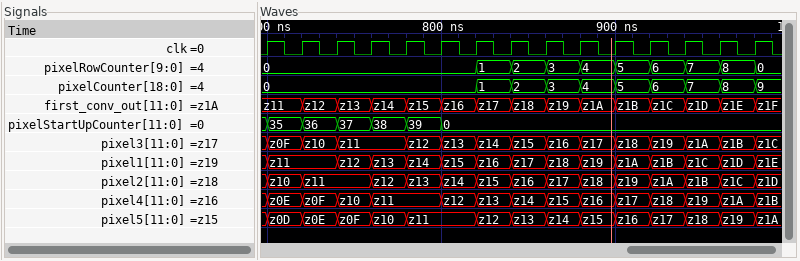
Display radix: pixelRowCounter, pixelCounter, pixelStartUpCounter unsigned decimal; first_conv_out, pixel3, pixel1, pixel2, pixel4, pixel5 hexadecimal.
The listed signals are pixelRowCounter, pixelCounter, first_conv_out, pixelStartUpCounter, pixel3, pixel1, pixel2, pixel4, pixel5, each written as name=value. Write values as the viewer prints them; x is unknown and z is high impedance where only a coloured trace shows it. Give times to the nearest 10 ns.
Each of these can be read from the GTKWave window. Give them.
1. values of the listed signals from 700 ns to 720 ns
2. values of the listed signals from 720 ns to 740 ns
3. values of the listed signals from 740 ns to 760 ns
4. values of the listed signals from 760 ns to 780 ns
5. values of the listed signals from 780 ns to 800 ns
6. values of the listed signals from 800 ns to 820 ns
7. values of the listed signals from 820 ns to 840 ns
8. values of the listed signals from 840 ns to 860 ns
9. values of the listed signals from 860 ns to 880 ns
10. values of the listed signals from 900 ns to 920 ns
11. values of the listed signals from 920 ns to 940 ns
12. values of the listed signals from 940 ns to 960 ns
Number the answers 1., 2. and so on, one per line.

1. pixelRowCounter=0, pixelCounter=0, first_conv_out=z11, pixelStartUpCounter=35, pixel3=z0F, pixel1=z11, pixel2=z10, pixel4=z0E, pixel5=z0D
2. pixelRowCounter=0, pixelCounter=0, first_conv_out=z12, pixelStartUpCounter=36, pixel3=z10, pixel1=z11, pixel2=z11, pixel4=z0F, pixel5=z0E
3. pixelRowCounter=0, pixelCounter=0, first_conv_out=z13, pixelStartUpCounter=37, pixel3=z11, pixel1=z12, pixel2=z11, pixel4=z10, pixel5=z0F
4. pixelRowCounter=0, pixelCounter=0, first_conv_out=z14, pixelStartUpCounter=38, pixel3=z11, pixel1=z13, pixel2=z12, pixel4=z11, pixel5=z10
5. pixelRowCounter=0, pixelCounter=0, first_conv_out=z15, pixelStartUpCounter=39, pixel3=z12, pixel1=z14, pixel2=z13, pixel4=z11, pixel5=z11
6. pixelRowCounter=0, pixelCounter=0, first_conv_out=z16, pixelStartUpCounter=0, pixel3=z13, pixel1=z15, pixel2=z14, pixel4=z12, pixel5=z11
7. pixelRowCounter=1, pixelCounter=1, first_conv_out=z17, pixelStartUpCounter=0, pixel3=z14, pixel1=z16, pixel2=z15, pixel4=z13, pixel5=z12
8. pixelRowCounter=2, pixelCounter=2, first_conv_out=z18, pixelStartUpCounter=0, pixel3=z15, pixel1=z17, pixel2=z16, pixel4=z14, pixel5=z13
9. pixelRowCounter=3, pixelCounter=3, first_conv_out=z19, pixelStartUpCounter=0, pixel3=z16, pixel1=z18, pixel2=z17, pixel4=z15, pixel5=z14
10. pixelRowCounter=5, pixelCounter=5, first_conv_out=z1B, pixelStartUpCounter=0, pixel3=z18, pixel1=z1A, pixel2=z19, pixel4=z17, pixel5=z16
11. pixelRowCounter=6, pixelCounter=6, first_conv_out=z1C, pixelStartUpCounter=0, pixel3=z19, pixel1=z1B, pixel2=z1A, pixel4=z18, pixel5=z17
12. pixelRowCounter=7, pixelCounter=7, first_conv_out=z1D, pixelStartUpCounter=0, pixel3=z1A, pixel1=z1C, pixel2=z1B, pixel4=z19, pixel5=z18
